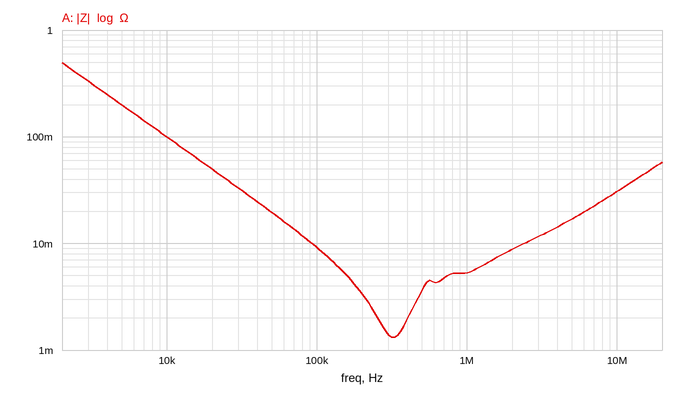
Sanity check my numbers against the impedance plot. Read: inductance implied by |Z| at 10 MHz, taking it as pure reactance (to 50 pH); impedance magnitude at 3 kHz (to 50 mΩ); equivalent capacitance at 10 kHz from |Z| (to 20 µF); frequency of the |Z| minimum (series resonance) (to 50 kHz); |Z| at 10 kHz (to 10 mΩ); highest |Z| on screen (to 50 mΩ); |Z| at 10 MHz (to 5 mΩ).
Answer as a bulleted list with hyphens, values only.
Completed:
- 500 pH
- 350 mΩ
- 160 µF
- 300 kHz
- 100 mΩ
- 500 mΩ
- 30 mΩ
